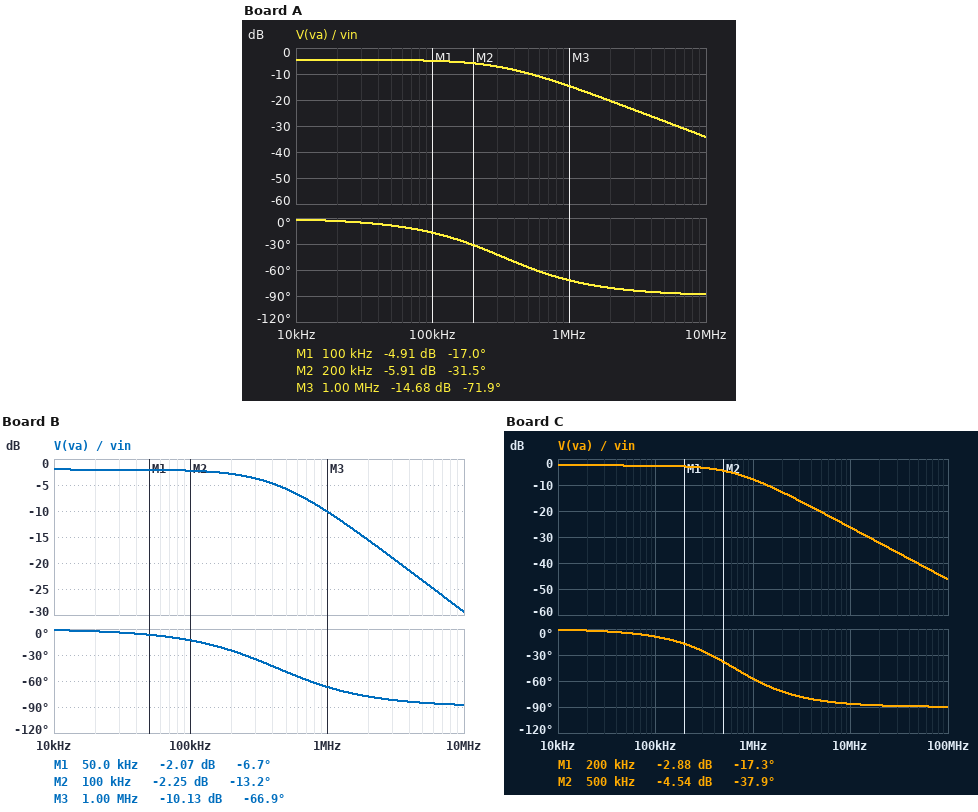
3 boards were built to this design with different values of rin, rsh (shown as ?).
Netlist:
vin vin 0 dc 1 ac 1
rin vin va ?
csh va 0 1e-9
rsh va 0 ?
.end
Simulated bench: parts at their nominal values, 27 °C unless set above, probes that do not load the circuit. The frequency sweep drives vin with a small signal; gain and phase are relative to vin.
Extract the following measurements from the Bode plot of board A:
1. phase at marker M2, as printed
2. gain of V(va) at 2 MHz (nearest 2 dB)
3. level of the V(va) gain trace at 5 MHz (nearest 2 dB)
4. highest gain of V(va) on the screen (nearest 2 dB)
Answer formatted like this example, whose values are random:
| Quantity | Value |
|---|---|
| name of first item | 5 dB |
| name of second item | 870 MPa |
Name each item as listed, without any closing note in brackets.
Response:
| Quantity | Value |
|---|---|
| phase at marker M2, as printed | -31.5 deg |
| gain of V(va) at 2 MHz | -20 dB |
| level of the V(va) gain trace at 5 MHz | -28 dB |
| highest gain of V(va) on the screen | -4 dB |
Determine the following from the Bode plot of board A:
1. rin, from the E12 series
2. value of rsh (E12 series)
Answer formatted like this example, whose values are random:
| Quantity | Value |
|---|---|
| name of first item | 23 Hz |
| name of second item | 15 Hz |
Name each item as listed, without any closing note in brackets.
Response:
| Quantity | Value |
|---|---|
| rin, from the E12 series | 820 Ω |
| value of rsh | 1.2 kΩ |
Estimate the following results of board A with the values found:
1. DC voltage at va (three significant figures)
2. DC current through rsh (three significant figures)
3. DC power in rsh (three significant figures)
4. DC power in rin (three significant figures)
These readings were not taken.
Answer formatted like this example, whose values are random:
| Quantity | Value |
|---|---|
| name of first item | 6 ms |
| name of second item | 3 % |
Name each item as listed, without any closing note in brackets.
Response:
| Quantity | Value |
|---|---|
| DC voltage at va | 594 mV |
| DC current through rsh | 495 µA |
| DC power in rsh | 294 µW |
| DC power in rin | 201 µW |
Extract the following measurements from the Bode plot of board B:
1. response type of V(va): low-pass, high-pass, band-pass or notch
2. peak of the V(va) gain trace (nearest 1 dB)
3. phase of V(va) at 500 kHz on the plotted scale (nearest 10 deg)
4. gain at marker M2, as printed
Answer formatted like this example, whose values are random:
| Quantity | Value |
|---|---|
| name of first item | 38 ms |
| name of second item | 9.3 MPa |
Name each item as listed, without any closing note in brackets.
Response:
| Quantity | Value |
|---|---|
| response type of V(va): low-pass, high-pass, band-pass or notch | low-pass |
| peak of the V(va) gain trace | -2 dB |
| phase of V(va) at 500 kHz on the plotted scale | -50 deg |
| gain at marker M2, as printed | -2.25 dB |
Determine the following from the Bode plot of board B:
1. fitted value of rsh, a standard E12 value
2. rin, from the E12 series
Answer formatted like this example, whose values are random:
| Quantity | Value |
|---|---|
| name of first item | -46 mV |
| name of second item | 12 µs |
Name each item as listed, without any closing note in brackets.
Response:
| Quantity | Value |
|---|---|
| fitted value of rsh, a standard E12 value | 1.8 kΩ |
| rin, from the E12 series | 470 Ω |
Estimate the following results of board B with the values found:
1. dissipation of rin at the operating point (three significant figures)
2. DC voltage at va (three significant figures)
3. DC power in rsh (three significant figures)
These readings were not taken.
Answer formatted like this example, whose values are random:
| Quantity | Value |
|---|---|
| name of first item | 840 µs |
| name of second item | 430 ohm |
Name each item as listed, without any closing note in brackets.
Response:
| Quantity | Value |
|---|---|
| dissipation of rin at the operating point | 91.2 µW |
| DC voltage at va | 793 mV |
| DC power in rsh | 349 µW |
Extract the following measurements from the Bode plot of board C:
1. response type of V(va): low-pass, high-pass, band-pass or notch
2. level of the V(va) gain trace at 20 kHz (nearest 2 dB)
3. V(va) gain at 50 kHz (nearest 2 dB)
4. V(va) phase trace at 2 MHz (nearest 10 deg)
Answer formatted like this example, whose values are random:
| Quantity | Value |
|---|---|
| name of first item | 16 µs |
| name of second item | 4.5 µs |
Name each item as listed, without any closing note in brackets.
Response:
| Quantity | Value |
|---|---|
| response type of V(va): low-pass, high-pass, band-pass or notch | low-pass |
| level of the V(va) gain trace at 20 kHz | -2 dB |
| V(va) gain at 50 kHz | -2 dB |
| V(va) phase trace at 2 MHz | -70 deg |
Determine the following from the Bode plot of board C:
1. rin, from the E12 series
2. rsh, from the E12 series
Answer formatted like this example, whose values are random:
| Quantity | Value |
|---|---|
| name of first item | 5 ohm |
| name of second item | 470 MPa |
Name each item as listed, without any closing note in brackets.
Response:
| Quantity | Value |
|---|---|
| rin, from the E12 series | 330 Ω |
| rsh, from the E12 series | 1 kΩ |
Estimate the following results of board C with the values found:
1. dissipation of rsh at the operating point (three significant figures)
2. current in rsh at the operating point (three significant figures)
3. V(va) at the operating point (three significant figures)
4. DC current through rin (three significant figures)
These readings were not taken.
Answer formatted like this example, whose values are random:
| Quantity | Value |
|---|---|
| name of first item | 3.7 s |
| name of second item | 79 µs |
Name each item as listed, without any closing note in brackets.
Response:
| Quantity | Value |
|---|---|
| dissipation of rsh at the operating point | 565 µW |
| current in rsh at the operating point | 752 µA |
| V(va) at the operating point | 752 mV |
| DC current through rin | 752 µA |
